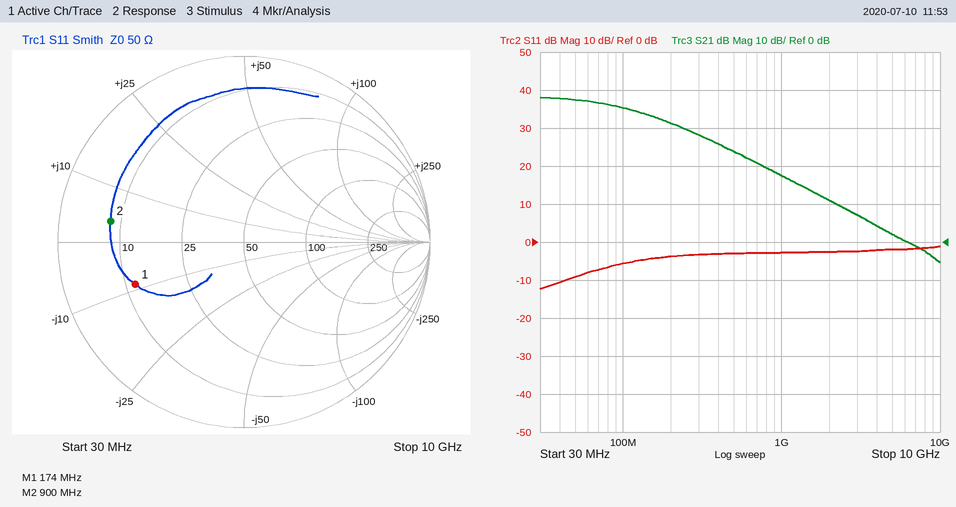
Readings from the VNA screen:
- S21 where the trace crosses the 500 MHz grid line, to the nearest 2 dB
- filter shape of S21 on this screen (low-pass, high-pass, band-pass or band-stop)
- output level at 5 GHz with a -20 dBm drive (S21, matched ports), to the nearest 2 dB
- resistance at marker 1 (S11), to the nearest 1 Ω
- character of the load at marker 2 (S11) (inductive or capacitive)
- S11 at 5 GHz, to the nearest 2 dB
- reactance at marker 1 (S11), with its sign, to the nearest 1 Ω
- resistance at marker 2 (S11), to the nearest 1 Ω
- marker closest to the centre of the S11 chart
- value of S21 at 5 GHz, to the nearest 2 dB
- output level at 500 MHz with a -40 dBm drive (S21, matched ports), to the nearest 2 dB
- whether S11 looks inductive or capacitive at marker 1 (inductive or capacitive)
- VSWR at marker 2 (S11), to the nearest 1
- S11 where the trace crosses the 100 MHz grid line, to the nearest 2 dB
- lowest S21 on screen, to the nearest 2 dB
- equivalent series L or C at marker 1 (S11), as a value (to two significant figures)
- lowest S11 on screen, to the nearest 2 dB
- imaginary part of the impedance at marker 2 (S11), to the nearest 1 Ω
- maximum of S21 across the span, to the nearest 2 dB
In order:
24 dB
low-pass
-18 dBm
12 Ω
inductive
-2 dB
-9 Ω
8 Ω
marker 1
2 dB
-16 dBm
capacitive
6
-6 dB
-6 dB
100 pF
-12 dB
+4 Ω
38 dB
